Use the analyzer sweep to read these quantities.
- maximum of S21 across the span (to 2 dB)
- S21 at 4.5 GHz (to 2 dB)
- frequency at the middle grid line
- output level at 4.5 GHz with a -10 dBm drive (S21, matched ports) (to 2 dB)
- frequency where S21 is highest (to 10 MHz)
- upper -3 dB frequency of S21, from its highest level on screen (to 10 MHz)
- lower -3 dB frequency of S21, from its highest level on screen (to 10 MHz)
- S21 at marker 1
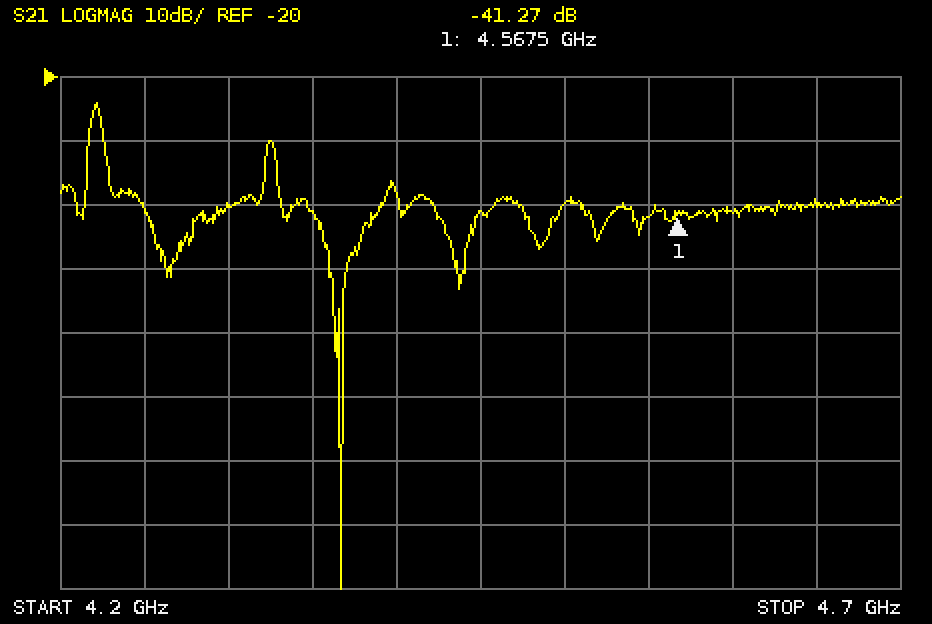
-24 dB
-40 dB
4.45 GHz
-50 dBm
4.22 GHz
4.22 GHz
4.22 GHz
-41.27 dB
